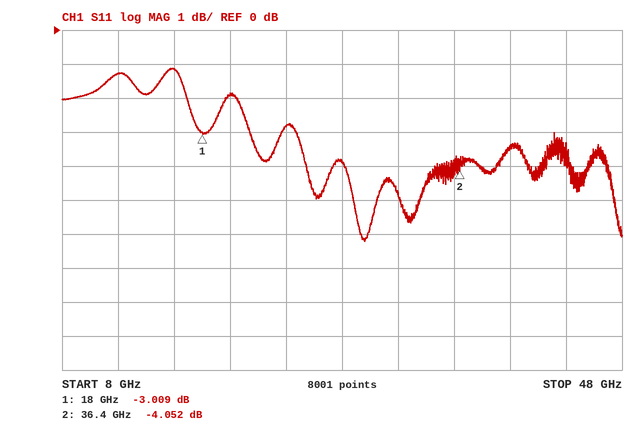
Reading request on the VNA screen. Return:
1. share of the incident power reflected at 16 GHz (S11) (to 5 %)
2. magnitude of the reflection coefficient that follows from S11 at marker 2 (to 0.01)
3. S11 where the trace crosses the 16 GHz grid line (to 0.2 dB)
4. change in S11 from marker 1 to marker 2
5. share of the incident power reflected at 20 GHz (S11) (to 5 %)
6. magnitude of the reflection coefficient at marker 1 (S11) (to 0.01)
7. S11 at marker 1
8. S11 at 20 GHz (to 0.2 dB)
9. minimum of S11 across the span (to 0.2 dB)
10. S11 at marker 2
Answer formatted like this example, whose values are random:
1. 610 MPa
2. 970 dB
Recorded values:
1. 75 %
2. 0.63
3. -1.2 dB
4. -1.043 dB
5. 65 %
6. 0.71
7. -3.009 dB
8. -2.0 dB
9. -6.2 dB
10. -4.052 dB
